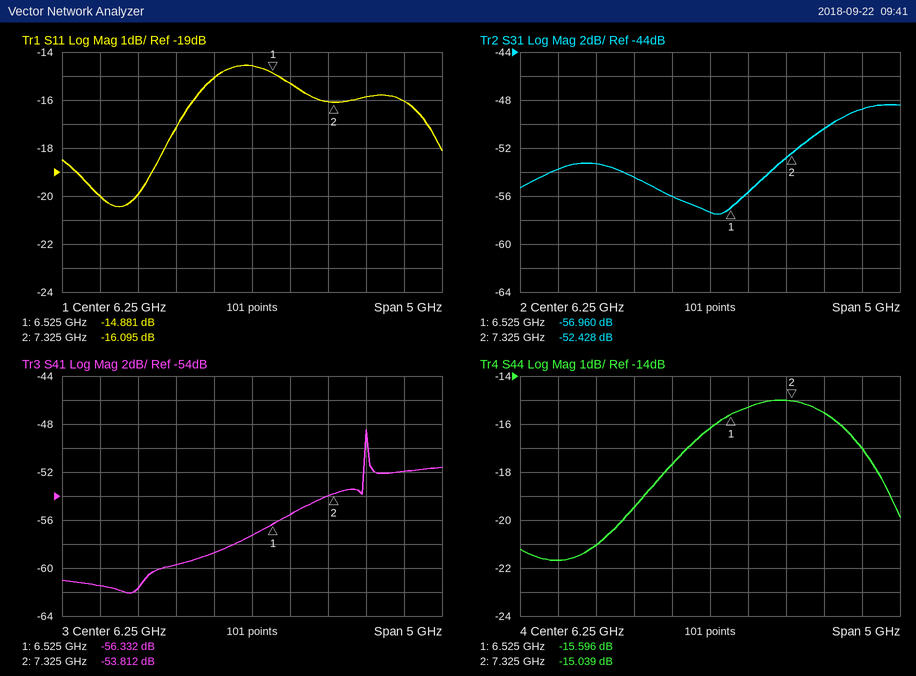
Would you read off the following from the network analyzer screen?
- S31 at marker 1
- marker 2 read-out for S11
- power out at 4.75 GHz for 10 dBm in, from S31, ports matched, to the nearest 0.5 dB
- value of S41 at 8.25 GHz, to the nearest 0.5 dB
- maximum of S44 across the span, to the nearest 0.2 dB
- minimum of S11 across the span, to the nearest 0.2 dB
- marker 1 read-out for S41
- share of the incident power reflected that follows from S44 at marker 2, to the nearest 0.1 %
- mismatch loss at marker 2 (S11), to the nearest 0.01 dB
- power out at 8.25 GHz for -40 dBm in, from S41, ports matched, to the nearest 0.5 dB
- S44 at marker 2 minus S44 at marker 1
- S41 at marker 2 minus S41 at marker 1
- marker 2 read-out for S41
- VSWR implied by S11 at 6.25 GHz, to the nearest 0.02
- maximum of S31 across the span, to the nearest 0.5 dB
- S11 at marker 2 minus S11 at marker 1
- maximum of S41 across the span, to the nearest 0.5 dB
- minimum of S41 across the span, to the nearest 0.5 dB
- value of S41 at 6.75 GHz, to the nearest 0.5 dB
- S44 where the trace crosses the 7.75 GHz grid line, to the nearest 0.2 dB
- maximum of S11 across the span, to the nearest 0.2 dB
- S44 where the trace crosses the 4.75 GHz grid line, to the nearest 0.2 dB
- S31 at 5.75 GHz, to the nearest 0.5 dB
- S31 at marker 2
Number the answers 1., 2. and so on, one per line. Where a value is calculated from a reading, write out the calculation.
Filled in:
1. -56.960 dB
2. -16.095 dB
3. 10 dBm + (-53.5 dB) = -43.5 dBm
4. -52.0 dB
5. -15.0 dB
6. -20.4 dB
7. -56.332 dB
8. 10^(-15.039/10) ≈ 3.1 %
9. −10 log10(1 − 10^(-16.095/10)) ≈ 0.11 dB
10. -40 dBm + (-52.0 dB) = -92.0 dBm
11. -15.039 − (-15.596) = 0.557 dB
12. -53.812 − (-56.332) = 2.520 dB
13. -53.812 dB
14. |Γ| = 10^(-14.6/20) = 0.1862; VSWR = (1 + 0.1862)/(1 − 0.1862) ≈ 1.46
15. -48.5 dB
16. -16.095 − (-14.881) = -1.214 dB
17. -48.5 dB
18. -62.0 dB
19. -55.5 dB
20. -15.6 dB
21. -14.6 dB
22. -21.0 dB
23. -56.0 dB
24. -52.428 dB
